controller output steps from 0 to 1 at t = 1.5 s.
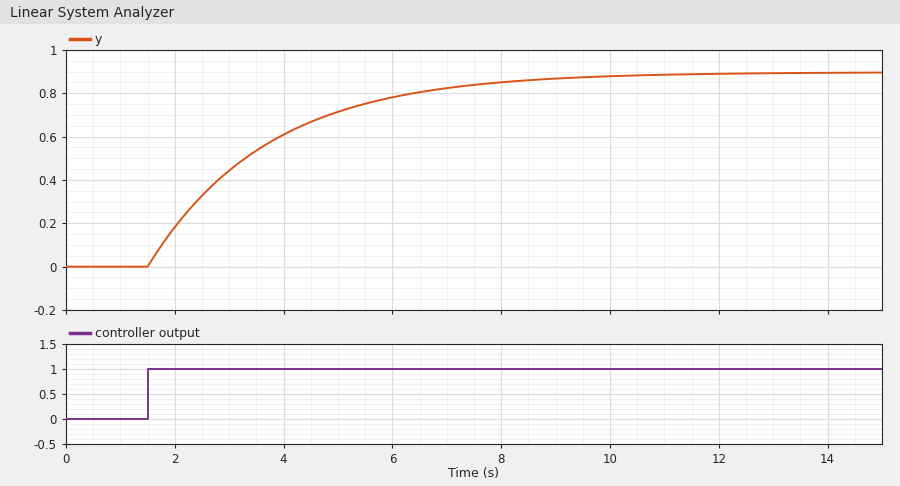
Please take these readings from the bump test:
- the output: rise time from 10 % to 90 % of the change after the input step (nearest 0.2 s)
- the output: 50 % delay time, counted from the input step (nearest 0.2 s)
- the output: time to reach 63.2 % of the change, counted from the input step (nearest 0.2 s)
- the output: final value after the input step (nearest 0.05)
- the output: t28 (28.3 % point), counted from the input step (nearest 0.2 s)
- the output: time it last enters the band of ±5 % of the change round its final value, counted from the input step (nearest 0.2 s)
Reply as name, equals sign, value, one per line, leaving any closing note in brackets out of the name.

the output: rise time from 10 % to 90 % of the change after the input step = 4.8 s
the output: 50 % delay time, counted from the input step = 1.6 s
the output: time to reach 63.2 % of the change, counted from the input step = 2.2 s
the output: final value after the input step = 0.90
the output: t28 (28.3 % point), counted from the input step = 0.8 s
the output: time it last enters the band of ±5 % of the change round its final value, counted from the input step = 6.6 s
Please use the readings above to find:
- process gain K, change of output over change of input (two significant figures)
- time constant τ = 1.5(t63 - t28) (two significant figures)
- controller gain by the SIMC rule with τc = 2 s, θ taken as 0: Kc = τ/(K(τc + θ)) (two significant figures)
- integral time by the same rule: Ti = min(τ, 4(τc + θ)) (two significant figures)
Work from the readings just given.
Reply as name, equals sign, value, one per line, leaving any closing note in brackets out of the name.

process gain K, change of output over change of input = 0.90
time constant τ = 1.5(t63 - t28) = 2.1 s
controller gain by the SIMC rule with τc = 2 s, θ taken as 0: Kc = τ/(K(τc + θ)) = 1.2
integral time by the same rule: Ti = min(τ, 4(τc + θ)) = 2.1 s
